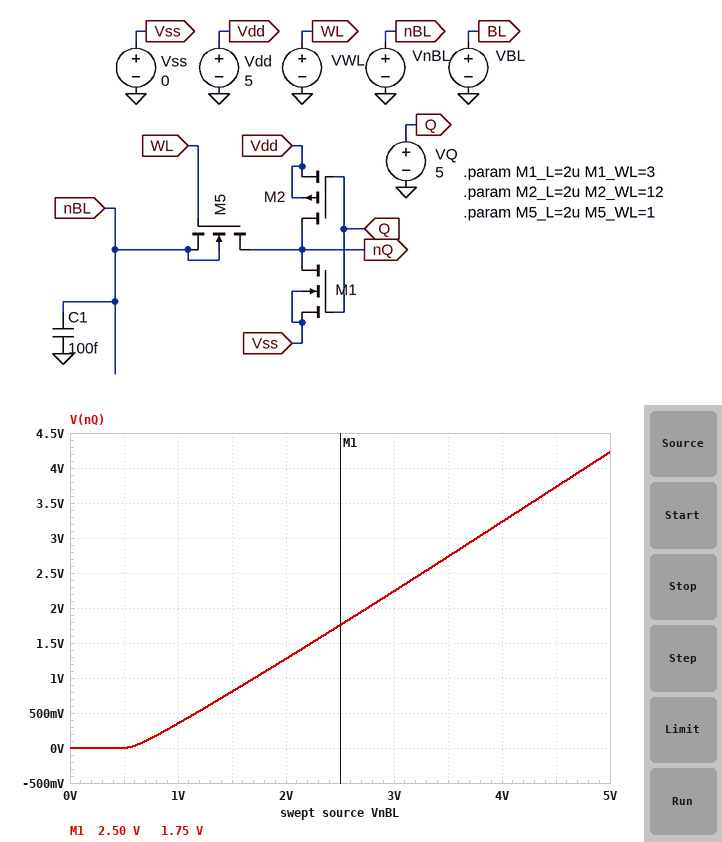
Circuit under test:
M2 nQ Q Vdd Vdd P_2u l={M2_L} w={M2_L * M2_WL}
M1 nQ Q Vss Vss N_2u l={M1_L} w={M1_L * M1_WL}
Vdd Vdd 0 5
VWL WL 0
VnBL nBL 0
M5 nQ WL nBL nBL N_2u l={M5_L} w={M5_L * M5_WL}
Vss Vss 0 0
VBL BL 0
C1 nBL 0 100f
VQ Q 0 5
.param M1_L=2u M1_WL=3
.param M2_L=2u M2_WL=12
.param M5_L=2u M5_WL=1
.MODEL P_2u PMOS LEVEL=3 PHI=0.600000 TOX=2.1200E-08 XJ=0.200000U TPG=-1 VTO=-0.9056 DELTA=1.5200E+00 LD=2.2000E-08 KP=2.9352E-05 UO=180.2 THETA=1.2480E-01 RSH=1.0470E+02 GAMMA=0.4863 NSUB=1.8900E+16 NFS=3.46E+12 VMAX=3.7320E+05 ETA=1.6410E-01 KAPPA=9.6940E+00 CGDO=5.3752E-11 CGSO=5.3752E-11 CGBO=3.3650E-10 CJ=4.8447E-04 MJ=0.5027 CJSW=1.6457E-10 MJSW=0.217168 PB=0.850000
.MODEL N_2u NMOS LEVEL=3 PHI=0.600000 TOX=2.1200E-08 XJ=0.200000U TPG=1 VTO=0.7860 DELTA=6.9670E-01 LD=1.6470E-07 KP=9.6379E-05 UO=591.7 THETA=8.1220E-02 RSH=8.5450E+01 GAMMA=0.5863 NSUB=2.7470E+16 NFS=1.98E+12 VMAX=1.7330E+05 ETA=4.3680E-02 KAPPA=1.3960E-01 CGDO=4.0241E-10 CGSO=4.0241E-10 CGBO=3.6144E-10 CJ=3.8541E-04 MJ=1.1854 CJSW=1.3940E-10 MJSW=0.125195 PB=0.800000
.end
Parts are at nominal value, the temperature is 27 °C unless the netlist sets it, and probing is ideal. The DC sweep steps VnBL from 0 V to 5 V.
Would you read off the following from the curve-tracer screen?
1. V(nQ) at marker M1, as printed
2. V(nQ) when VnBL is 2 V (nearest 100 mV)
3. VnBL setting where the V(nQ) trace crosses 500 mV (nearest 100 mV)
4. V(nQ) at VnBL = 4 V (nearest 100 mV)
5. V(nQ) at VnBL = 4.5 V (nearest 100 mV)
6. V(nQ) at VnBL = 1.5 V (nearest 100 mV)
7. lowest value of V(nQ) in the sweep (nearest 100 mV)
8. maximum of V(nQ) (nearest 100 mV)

1.75 V
1.3 V
1.2 V
3.2 V
3.7 V
800 mV
0 V
4.2 V
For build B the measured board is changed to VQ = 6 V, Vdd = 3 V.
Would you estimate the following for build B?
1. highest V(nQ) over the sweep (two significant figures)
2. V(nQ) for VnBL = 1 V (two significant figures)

3.9 V
340 mV
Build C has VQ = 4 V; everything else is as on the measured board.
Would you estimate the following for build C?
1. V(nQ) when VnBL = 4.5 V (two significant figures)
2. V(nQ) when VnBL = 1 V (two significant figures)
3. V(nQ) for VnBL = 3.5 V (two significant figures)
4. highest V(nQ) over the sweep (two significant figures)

3.8 V
360 mV
2.8 V
4.3 V
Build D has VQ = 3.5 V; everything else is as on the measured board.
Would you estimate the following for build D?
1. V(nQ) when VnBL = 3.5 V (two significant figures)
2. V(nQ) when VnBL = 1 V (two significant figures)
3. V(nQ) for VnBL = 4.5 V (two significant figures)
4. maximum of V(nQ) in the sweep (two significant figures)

2.8 V
380 mV
3.8 V
4.3 V
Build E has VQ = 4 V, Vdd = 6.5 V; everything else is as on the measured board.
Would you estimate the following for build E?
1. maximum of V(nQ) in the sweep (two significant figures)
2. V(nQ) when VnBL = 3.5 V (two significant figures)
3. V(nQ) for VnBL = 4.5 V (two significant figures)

4.3 V
2.8 V
3.8 V
